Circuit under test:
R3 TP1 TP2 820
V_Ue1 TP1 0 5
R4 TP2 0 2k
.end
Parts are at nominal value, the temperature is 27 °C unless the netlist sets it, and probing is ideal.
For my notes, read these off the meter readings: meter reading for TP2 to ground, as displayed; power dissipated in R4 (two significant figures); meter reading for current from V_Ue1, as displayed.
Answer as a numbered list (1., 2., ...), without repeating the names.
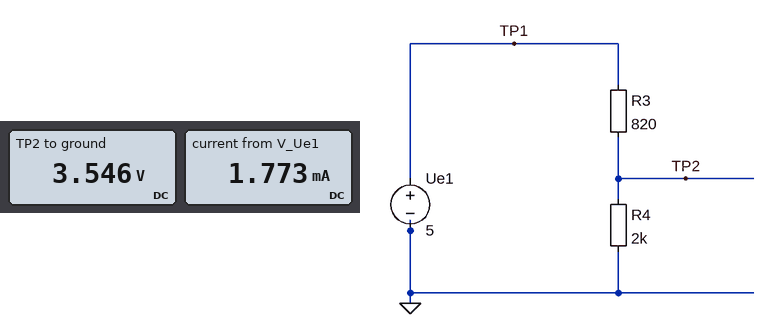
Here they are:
1. 3.546 V
2. 6.3 mW
3. 1.773 mA
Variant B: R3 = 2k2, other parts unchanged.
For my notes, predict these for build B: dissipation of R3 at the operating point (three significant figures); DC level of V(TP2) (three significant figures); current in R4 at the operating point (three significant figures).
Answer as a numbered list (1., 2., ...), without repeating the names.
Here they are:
1. 3.12 mW
2. 2.38 V
3. 1.19 mA
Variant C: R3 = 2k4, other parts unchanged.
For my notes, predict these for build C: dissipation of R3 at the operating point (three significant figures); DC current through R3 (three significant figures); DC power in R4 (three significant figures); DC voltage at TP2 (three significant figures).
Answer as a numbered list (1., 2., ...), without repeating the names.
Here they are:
1. 3.10 mW
2. 1.14 mA
3. 2.58 mW
4. 2.27 V
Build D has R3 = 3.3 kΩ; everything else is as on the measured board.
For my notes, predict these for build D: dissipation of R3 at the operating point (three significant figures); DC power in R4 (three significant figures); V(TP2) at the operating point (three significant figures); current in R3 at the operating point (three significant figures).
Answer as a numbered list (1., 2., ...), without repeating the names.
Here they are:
1. 2.94 mW
2. 1.78 mW
3. 1.89 V
4. 943 µA
